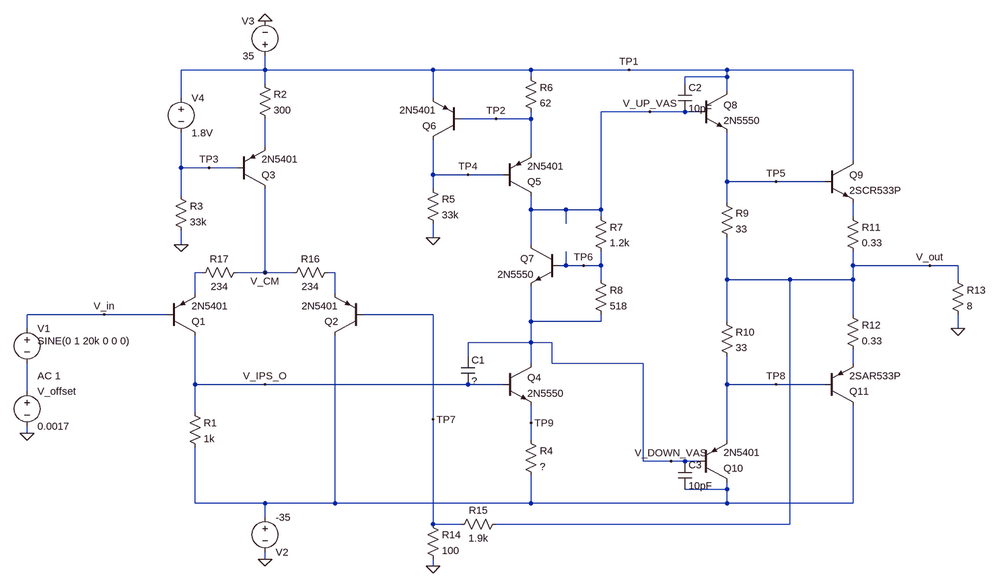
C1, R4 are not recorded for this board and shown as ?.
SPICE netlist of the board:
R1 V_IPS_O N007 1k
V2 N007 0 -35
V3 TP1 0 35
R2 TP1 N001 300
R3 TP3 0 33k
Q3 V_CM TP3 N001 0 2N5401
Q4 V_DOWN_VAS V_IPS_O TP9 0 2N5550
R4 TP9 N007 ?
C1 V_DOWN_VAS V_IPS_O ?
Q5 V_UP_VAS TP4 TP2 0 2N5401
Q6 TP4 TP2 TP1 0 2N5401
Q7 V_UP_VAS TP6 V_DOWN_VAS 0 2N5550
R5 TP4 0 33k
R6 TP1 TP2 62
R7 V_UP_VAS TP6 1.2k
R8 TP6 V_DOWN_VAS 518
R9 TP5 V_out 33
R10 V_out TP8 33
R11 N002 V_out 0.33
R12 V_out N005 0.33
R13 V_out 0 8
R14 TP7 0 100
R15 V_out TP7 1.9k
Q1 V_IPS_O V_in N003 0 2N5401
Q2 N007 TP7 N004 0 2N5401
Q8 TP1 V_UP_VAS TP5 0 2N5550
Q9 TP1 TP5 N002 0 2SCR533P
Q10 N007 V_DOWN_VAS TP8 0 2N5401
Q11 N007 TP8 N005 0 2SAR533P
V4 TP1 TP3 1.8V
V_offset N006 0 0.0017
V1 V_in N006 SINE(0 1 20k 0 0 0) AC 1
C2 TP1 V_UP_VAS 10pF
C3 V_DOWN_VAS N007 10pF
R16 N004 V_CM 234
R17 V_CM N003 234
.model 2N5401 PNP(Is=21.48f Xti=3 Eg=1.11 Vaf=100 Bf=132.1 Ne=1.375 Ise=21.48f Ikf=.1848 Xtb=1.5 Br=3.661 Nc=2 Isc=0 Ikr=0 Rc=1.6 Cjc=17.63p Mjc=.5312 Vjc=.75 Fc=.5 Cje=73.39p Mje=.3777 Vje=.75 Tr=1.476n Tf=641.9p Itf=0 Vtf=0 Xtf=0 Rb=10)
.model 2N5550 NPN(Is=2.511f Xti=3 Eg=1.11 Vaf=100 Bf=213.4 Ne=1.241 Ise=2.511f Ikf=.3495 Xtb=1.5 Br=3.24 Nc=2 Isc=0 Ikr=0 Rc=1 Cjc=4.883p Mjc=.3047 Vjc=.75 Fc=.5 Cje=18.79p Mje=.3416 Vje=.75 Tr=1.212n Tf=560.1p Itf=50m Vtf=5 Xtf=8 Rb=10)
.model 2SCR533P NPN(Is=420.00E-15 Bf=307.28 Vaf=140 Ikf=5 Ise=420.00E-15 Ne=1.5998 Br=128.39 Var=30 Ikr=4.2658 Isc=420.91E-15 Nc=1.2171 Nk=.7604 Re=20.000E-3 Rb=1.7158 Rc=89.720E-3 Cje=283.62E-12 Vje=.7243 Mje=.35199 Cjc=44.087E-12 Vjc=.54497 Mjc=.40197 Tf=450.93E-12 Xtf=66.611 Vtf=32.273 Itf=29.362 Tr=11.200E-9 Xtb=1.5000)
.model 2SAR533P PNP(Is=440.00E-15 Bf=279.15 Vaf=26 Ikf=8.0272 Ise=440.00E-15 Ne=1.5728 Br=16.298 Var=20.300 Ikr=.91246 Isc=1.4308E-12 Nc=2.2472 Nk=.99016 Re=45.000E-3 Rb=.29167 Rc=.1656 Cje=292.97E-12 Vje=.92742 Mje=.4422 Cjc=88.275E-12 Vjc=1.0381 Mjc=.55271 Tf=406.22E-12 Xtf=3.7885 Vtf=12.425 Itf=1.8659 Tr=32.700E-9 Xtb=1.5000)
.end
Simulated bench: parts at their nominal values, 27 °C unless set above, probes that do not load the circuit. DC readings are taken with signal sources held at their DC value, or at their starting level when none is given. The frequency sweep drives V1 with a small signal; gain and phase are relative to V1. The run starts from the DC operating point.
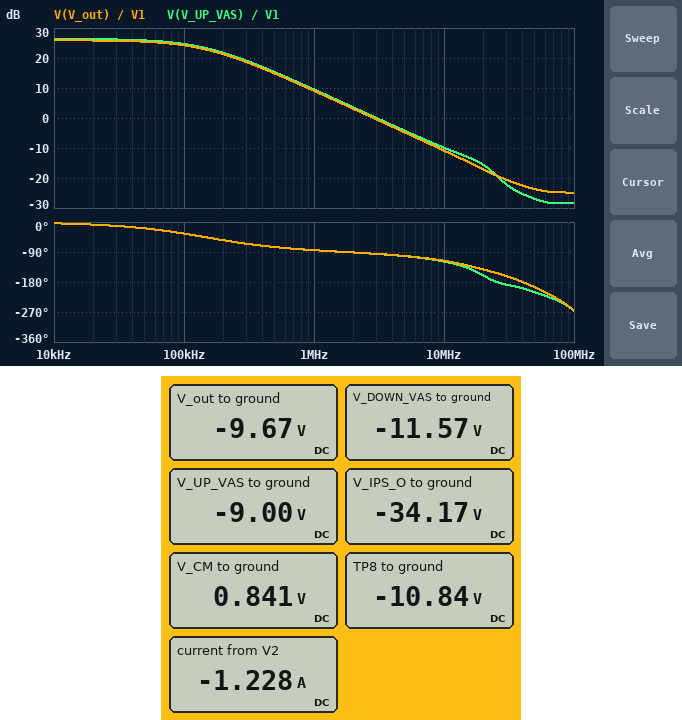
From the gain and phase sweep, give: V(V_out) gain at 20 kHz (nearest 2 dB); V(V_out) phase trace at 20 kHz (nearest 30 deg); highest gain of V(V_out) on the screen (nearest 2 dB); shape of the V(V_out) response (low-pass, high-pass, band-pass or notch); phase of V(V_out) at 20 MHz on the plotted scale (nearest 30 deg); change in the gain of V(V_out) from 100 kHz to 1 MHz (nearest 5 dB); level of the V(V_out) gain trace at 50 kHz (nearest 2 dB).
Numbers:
26 dB
0 deg
26 dB
low-pass
-150 deg
-15 dB
26 dB
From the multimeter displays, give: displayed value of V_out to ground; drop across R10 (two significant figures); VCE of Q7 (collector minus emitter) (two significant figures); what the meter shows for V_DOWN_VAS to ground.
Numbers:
-9.67 V
1.2 V
2.6 V
-11.57 V
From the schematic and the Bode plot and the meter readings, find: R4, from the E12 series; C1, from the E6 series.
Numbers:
8.2 Ω
100 pF
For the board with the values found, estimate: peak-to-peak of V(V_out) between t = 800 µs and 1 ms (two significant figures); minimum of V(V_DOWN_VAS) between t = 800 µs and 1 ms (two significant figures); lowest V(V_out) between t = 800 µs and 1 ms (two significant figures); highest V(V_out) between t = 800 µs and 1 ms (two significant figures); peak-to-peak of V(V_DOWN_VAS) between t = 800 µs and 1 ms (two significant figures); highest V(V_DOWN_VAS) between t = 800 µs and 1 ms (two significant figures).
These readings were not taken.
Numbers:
39 V
-32 V
-29 V
9.9 V
41 V
9.3 V
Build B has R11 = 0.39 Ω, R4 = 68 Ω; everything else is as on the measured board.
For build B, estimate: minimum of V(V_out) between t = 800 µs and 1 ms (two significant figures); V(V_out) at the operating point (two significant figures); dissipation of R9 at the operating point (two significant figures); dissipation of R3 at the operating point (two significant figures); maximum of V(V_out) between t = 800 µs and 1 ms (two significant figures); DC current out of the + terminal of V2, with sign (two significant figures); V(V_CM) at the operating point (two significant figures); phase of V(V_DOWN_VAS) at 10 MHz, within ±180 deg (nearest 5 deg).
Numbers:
-23 V
-3.5 V
2.0 mW
33 mW
16 V
-460 mA
1.0 V
-140 deg
